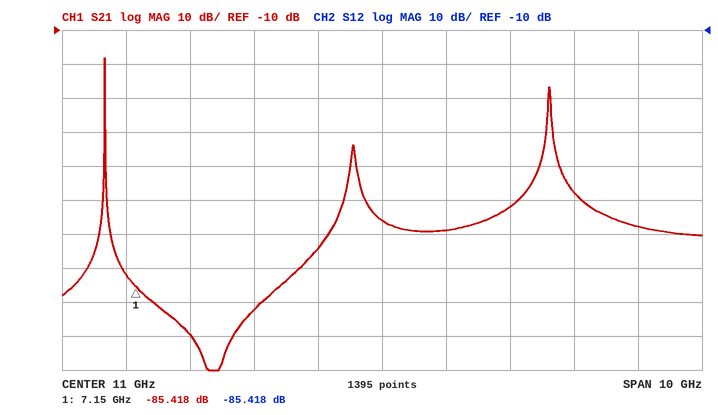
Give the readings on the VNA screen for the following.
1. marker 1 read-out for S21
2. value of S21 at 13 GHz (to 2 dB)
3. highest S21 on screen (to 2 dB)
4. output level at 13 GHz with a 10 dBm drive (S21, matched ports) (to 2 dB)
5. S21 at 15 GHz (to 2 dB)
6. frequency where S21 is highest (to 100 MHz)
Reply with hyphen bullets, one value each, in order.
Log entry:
- -85.418 dB
- -62 dB
- -18 dB
- -52 dBm
- -68 dB
- 6.7 GHz
